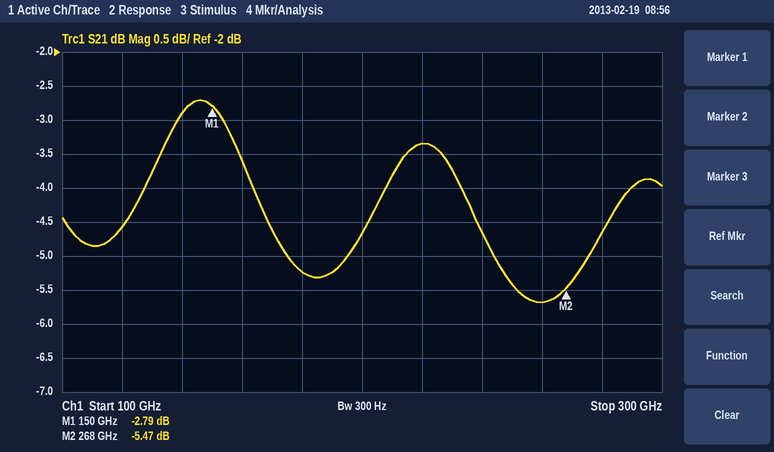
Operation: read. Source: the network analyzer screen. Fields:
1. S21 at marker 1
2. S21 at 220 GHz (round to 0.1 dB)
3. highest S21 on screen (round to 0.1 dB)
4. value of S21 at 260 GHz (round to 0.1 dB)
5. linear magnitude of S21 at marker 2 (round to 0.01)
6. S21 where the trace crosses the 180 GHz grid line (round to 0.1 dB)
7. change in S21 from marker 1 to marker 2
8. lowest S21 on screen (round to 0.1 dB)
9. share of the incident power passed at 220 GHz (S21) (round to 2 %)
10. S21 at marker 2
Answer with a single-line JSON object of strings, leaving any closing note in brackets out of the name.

{"S21 at marker 1": "-2.79 dB", "S21 at 220 GHz": "-3.3 dB", "highest S21 on screen": "-2.7 dB", "value of S21 at 260 GHz": "-5.7 dB", "linear magnitude of S21 at marker 2": "0.53", "S21 where the trace crosses the 180 GHz grid line": "-5.2 dB", "change in S21 from marker 1 to marker 2": "-2.68 dB", "lowest S21 on screen": "-5.7 dB", "share of the incident power passed at 220 GHz (S21)": "46 %", "S21 at marker 2": "-5.47 dB"}
